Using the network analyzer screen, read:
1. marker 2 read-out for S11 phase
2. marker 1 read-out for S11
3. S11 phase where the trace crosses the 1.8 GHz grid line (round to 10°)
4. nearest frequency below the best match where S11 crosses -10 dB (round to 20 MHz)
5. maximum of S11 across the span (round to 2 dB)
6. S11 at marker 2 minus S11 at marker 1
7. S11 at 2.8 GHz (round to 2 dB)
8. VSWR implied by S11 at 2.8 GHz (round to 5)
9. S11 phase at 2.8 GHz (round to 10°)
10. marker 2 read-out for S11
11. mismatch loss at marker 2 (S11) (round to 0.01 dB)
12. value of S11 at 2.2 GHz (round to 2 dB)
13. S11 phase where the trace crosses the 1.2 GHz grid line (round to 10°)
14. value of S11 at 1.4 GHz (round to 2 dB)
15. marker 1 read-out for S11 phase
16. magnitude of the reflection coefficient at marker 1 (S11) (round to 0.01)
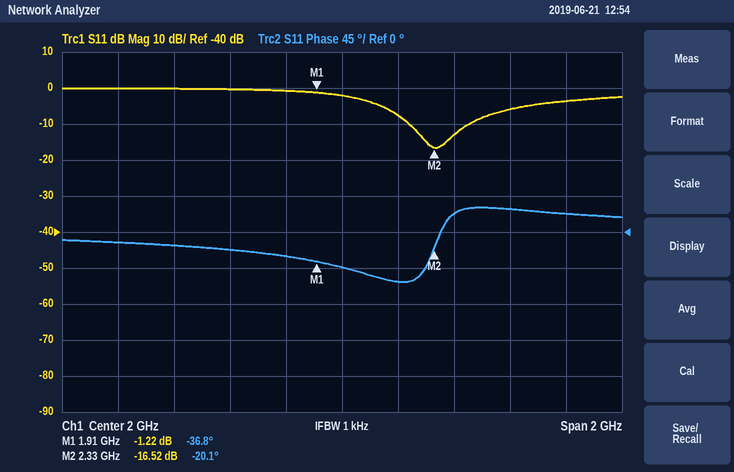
-20.1°
-1.22 dB
-30°
2.24 GHz
0 dB
-15.30 dB
-4 dB
5
20°
-16.52 dB
0.10 dB
-8 dB
-10°
0 dB
-36.8°
0.87
